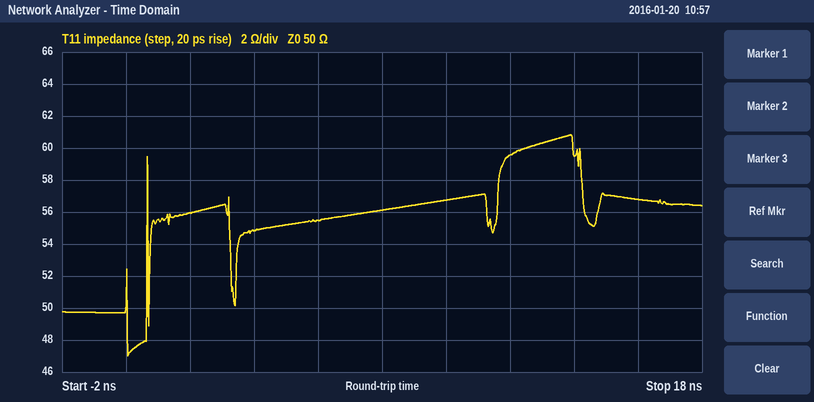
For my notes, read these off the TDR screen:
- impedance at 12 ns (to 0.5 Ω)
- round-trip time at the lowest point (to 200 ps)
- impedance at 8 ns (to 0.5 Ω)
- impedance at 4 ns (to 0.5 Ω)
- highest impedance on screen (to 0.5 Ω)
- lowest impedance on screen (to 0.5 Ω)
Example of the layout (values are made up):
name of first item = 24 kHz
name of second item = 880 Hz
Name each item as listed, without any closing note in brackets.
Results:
impedance at 12 ns = 59.5 Ω
round-trip time at the lowest point = 0.0 ns
impedance at 8 ns = 56.0 Ω
impedance at 4 ns = 55.0 Ω
highest impedance on screen = 61.0 Ω
lowest impedance on screen = 47.0 Ω
